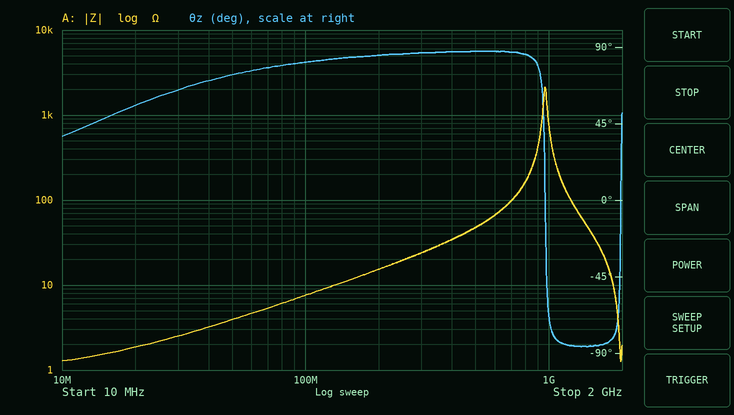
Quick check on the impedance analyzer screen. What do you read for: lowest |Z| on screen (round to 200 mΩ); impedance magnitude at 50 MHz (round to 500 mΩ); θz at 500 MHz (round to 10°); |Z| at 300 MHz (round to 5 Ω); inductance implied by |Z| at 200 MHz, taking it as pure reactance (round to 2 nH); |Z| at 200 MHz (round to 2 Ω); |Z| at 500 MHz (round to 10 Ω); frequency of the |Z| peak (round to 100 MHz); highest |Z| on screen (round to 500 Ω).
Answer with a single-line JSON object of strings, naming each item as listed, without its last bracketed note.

{"lowest |Z| on screen": "1.2 Ω", "impedance magnitude at 50 MHz": "4.0 Ω", "θz at 500 MHz": "90°", "|Z| at 300 MHz": "25 Ω", "inductance implied by |Z| at 200 MHz, taking it as pure reactance": "12 nH", "|Z| at 200 MHz": "16 Ω", "|Z| at 500 MHz": "50 Ω", "frequency of the |Z| peak": "1.0 GHz", "highest |Z| on screen": "2.0 kΩ"}
